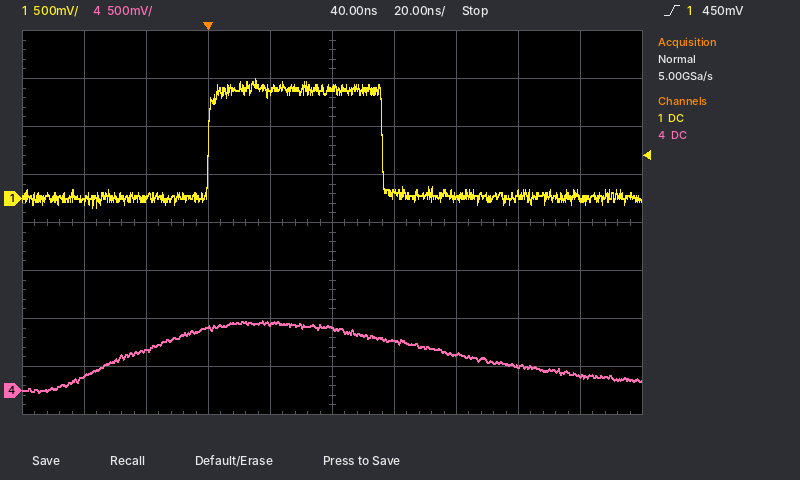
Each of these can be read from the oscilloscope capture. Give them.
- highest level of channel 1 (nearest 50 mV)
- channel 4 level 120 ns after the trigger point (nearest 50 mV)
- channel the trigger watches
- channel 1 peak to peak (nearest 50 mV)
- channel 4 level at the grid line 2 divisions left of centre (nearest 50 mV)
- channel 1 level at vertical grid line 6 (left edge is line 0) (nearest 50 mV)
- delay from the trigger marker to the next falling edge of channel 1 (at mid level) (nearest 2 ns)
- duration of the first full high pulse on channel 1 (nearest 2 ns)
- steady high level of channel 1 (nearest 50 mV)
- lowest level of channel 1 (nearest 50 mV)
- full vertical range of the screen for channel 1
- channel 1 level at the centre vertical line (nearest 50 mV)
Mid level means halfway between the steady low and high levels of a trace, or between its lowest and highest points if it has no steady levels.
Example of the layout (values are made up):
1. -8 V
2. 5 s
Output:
1. 1.25 V
2. 150 mV
3. channel 1
4. 1.35 V
5. 650 mV
6. 50 mV
7. 56 ns
8. 56 ns
9. 1.15 V
10. -100 mV
11. 4 V
12. 1.15 V
